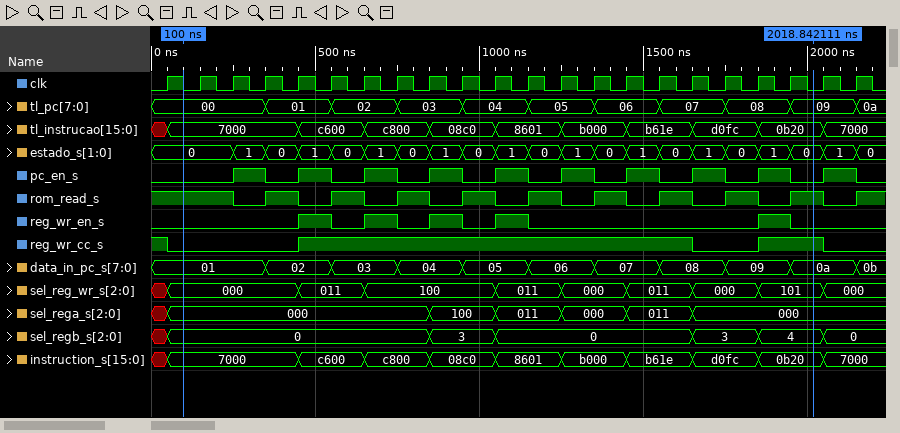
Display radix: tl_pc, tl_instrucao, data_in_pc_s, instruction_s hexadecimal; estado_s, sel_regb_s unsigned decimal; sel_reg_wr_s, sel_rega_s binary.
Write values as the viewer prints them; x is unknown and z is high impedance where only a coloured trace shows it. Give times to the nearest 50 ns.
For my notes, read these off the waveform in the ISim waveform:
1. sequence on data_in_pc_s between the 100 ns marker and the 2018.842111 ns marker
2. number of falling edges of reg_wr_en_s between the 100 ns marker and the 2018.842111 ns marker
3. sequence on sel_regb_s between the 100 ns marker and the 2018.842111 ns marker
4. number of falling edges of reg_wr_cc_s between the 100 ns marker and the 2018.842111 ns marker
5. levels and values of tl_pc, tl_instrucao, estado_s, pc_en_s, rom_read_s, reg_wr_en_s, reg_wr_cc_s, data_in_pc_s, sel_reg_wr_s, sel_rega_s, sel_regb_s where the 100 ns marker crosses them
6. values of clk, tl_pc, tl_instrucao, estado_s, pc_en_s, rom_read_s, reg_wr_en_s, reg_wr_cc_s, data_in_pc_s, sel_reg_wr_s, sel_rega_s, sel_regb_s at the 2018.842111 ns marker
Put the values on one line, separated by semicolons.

01, 02, 03, 04, 05, 06, 07, 08, 09, 0a; 5; 0, 3, 0, 3, 4; 1; tl_pc=00, tl_instrucao=7000, estado_s=0, pc_en_s=0, rom_read_s=1, reg_wr_en_s=0, reg_wr_cc_s=0, data_in_pc_s=01, sel_reg_wr_s=000, sel_rega_s=000, sel_regb_s=0; clk=0, tl_pc=09, tl_instrucao=0b20, estado_s=0, pc_en_s=0, rom_read_s=1, reg_wr_en_s=0, reg_wr_cc_s=1, data_in_pc_s=0a, sel_reg_wr_s=101, sel_rega_s=000, sel_regb_s=4
